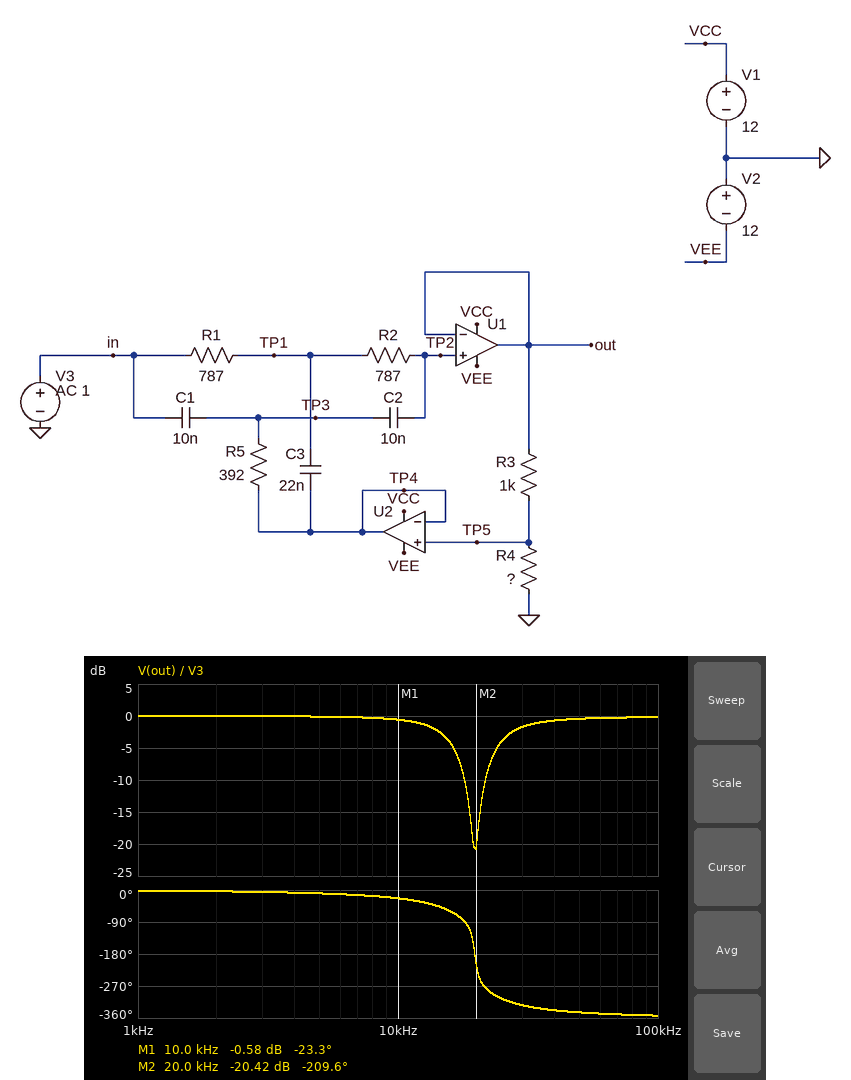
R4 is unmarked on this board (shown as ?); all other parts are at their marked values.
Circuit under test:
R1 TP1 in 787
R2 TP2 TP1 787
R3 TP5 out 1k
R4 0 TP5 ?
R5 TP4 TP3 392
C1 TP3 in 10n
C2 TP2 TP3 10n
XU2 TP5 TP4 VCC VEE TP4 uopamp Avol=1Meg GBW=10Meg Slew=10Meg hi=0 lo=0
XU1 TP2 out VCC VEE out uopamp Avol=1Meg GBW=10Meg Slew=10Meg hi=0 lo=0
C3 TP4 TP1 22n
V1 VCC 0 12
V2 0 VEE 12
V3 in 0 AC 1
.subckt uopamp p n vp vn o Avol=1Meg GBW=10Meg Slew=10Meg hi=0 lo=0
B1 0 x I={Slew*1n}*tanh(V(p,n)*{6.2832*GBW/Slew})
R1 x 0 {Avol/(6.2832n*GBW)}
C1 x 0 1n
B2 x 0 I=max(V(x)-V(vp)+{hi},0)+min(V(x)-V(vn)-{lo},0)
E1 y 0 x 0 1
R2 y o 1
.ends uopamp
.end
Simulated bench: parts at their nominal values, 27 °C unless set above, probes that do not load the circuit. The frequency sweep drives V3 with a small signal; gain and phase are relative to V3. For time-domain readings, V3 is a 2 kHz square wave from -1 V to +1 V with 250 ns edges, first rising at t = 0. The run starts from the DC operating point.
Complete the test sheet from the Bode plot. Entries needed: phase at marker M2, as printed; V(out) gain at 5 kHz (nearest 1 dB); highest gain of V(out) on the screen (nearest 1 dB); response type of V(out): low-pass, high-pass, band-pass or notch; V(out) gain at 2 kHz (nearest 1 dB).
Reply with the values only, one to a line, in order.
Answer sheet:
-209.6 deg
0 dB
0 dB
notch
0 dB
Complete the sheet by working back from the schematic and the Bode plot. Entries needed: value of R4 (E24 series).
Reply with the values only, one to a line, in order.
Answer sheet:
5.6 kΩ
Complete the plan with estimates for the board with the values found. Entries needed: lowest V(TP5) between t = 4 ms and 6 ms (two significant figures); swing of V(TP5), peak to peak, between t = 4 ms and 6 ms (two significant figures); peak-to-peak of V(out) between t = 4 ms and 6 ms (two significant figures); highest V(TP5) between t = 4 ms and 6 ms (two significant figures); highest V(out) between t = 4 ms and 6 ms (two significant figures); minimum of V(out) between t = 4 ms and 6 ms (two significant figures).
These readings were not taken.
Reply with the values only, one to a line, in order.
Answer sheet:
-1.1 V
2.3 V
2.7 V
1.1 V
1.3 V
-1.3 V
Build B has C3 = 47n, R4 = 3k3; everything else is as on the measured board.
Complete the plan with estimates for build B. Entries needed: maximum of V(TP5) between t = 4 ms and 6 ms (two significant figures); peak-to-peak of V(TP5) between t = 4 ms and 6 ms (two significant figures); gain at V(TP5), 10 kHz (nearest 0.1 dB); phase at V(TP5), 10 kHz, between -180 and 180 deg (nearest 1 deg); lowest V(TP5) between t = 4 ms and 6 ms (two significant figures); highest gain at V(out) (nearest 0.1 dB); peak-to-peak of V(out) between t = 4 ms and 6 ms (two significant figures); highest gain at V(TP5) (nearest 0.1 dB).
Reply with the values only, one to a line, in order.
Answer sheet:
1.0 V
2.0 V
-4.4 dB
-62 deg
-1.0 V
0 dB
2.6 V
-2.3 dB
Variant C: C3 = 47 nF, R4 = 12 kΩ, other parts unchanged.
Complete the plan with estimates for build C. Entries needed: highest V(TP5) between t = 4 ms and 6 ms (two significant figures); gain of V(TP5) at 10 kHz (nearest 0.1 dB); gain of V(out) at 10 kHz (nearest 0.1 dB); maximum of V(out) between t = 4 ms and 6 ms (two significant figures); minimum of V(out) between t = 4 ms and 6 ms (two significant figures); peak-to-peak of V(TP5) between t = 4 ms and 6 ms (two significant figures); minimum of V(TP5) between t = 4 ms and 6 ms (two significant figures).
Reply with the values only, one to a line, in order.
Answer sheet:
1.4 V
-0.1 dB
0.6 dB
1.5 V
-1.5 V
2.7 V
-1.4 V
